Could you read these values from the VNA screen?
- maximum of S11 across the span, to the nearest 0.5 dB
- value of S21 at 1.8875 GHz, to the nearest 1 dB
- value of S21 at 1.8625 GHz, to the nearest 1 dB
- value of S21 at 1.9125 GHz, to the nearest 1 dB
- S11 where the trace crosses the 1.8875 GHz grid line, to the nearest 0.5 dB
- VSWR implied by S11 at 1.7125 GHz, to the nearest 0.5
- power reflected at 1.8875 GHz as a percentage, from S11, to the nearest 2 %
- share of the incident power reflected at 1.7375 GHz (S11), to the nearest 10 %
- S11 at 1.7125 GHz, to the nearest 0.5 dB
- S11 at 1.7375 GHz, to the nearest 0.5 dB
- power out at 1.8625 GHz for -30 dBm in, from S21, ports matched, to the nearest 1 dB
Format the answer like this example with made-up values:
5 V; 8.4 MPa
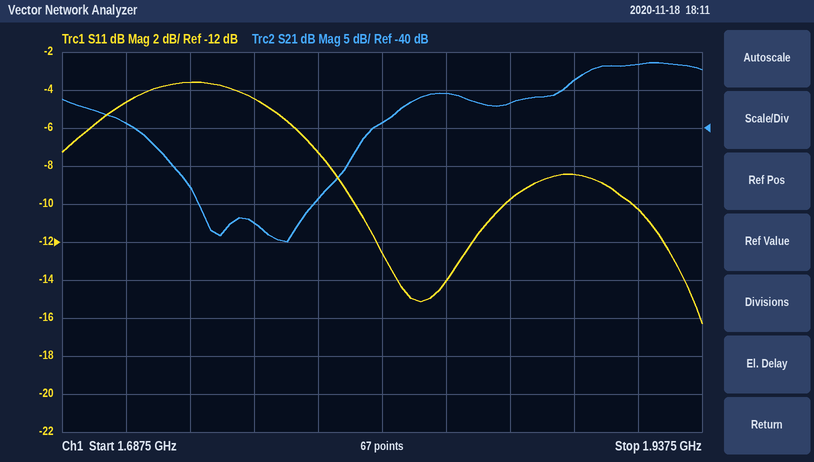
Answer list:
-3.5 dB; -34 dB; -37 dB; -32 dB; -8.5 dB; 4.0; 14 %; 40 %; -4.5 dB; -3.5 dB; -67 dBm
